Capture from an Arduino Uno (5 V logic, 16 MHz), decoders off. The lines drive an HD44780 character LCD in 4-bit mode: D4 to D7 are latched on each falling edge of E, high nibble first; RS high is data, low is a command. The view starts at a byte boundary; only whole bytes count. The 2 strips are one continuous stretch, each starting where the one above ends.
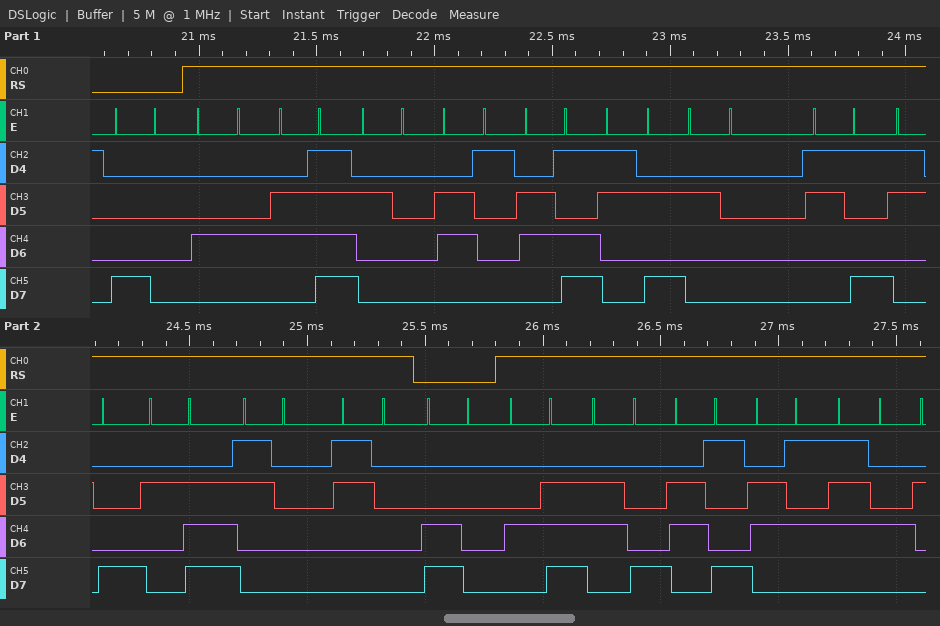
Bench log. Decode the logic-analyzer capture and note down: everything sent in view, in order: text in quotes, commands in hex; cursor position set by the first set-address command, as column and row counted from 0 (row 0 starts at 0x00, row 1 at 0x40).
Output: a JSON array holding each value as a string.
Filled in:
["0x80 \"Do am: 98.00\" 0xC0 \"Nhiet\"", "column 0, row 0"]
